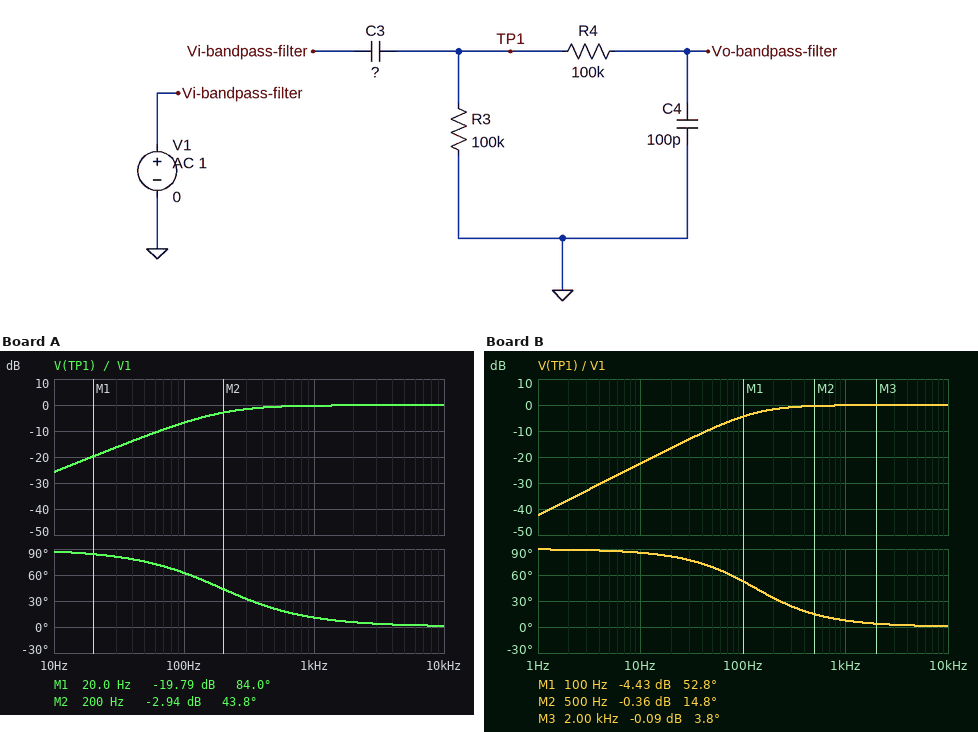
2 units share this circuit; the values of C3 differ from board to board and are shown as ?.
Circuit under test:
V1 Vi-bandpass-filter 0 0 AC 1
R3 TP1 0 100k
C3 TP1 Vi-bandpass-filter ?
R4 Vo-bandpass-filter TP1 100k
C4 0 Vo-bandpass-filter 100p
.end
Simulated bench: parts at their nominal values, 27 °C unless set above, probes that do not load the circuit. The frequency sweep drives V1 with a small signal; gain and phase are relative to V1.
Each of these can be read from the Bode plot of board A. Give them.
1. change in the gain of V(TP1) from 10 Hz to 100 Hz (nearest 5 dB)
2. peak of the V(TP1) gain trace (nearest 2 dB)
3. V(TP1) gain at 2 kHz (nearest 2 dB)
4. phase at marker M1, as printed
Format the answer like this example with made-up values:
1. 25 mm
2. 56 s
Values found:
1. 20 dB
2. 0 dB
3. 0 dB
4. 84.0 deg
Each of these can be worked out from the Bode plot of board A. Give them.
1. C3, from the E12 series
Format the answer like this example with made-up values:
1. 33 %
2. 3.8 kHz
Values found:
1. 8.2 nF
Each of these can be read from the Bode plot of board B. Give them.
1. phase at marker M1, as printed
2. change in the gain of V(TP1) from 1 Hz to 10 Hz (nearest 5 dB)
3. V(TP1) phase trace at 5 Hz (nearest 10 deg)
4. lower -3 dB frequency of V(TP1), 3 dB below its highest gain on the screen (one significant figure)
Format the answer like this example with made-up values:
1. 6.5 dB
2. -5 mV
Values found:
1. 52.8 deg
2. 20 dB
3. 90 deg
4. 100 Hz
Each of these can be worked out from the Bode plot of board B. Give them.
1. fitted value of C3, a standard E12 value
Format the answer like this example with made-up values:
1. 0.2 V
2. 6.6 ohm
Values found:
1. 12 nF
